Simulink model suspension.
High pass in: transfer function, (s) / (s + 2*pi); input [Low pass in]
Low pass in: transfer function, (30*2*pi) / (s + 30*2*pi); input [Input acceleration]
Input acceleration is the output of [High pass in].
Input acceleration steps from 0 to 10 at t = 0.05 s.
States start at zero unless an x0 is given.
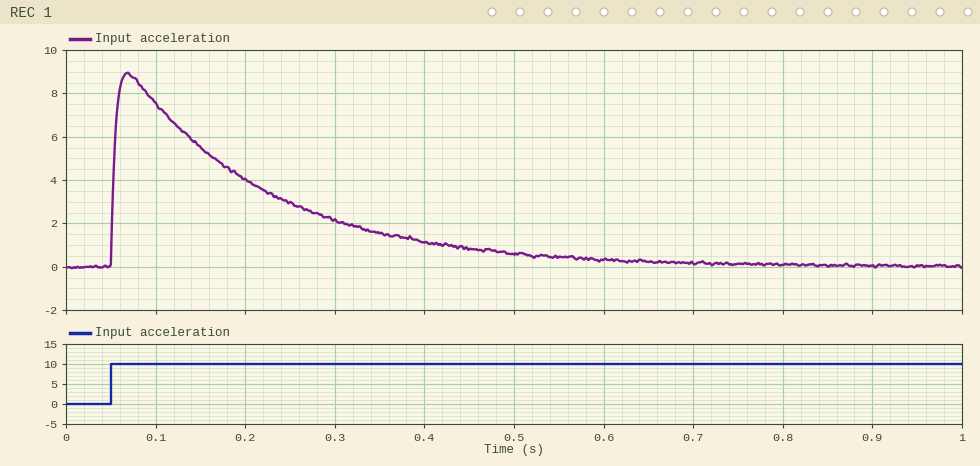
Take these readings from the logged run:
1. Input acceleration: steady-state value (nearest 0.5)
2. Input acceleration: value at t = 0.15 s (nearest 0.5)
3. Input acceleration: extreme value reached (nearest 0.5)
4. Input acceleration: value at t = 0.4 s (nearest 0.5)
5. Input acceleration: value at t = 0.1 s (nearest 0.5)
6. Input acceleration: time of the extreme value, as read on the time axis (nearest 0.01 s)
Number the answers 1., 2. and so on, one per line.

1. 0.0
2. 5.5
3. 9.0
4. 1.0
5. 7.5
6. 0.07 s
